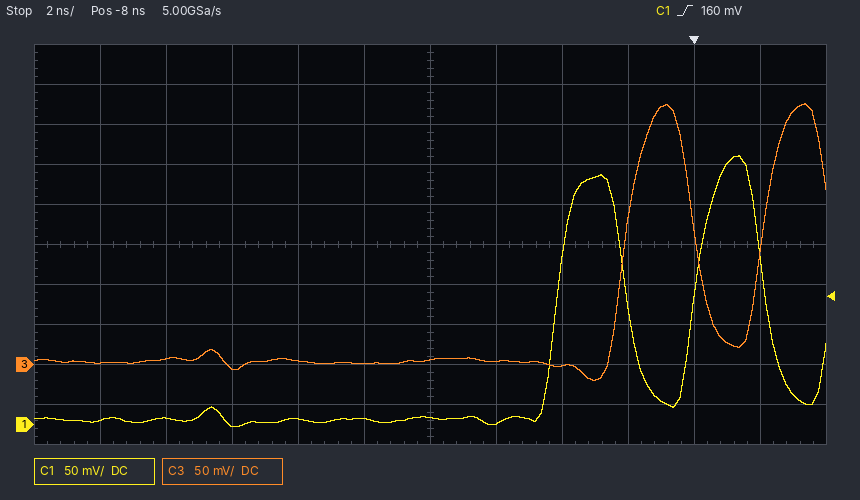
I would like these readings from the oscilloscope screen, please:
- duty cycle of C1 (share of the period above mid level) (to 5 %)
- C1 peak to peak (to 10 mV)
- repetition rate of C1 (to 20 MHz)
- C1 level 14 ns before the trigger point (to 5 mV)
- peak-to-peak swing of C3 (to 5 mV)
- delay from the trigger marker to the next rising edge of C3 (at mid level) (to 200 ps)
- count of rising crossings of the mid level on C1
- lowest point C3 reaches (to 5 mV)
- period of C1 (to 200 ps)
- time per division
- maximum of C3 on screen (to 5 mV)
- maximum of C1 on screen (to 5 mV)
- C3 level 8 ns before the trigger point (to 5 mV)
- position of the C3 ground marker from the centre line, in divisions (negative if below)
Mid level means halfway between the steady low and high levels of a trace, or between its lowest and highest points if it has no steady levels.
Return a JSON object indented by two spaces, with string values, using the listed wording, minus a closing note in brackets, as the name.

{
  "duty cycle of C1 (share of the period above mid level)": "50 %",
  "C1 peak to peak": "340 mV",
  "repetition rate of C1": "240 MHz",
  "C1 level 14 ns before the trigger point": "0 mV",
  "peak-to-peak swing of C3": "345 mV",
  "delay from the trigger marker to the next rising edge of C3 (at mid level)": "2.0 ns",
  "count of rising crossings of the mid level on C1": "2",
  "lowest point C3 reaches": "-20 mV",
  "period of C1": "4.2 ns",
  "time per division": "2 ns",
  "maximum of C3 on screen": "325 mV",
  "maximum of C1 on screen": "335 mV",
  "C3 level 8 ns before the trigger point": "5 mV",
  "position of the C3 ground marker from the centre line, in divisions": "-3.0 div"
}
